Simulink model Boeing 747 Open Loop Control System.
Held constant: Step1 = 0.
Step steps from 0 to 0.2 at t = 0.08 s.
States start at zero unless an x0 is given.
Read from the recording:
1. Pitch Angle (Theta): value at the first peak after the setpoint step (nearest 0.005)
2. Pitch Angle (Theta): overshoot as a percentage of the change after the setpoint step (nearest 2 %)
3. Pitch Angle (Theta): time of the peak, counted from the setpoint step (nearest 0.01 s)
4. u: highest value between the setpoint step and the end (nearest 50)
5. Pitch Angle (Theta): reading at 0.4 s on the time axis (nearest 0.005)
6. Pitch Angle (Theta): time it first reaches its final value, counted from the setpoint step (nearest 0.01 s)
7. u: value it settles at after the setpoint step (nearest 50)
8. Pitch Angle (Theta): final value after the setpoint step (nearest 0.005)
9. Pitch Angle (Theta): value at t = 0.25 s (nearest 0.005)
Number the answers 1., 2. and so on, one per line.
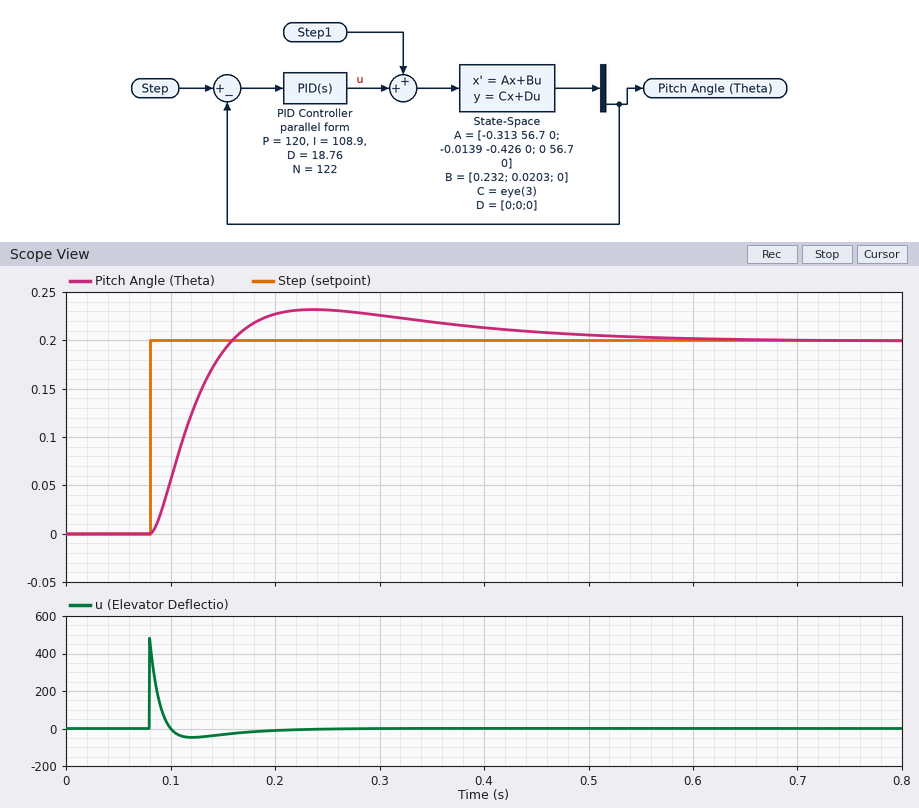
1. 0.230
2. 16 %
3. 0.16 s
4. 500
5. 0.215
6. 0.08 s
7. 0
8. 0.200
9. 0.230
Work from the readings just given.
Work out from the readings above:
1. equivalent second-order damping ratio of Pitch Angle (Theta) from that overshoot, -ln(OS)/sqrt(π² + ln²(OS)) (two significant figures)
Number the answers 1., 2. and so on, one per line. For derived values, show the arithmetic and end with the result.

1. ln(0.16) = -1.833; 1.833 / sqrt(9.870 + 3.358) = 0.50
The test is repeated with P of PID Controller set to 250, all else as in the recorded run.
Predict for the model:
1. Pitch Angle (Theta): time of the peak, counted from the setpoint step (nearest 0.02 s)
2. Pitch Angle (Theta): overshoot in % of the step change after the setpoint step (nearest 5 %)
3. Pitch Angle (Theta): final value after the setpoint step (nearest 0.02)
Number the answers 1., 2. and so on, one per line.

1. 0.12 s
2. 25 %
3. 0.20
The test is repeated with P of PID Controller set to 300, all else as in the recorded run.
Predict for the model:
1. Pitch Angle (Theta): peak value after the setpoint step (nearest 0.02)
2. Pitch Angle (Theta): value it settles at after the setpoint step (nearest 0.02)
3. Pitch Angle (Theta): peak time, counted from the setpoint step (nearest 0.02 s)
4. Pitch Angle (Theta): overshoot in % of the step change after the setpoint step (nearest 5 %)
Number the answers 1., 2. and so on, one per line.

1. 0.26
2. 0.20
3. 0.12 s
4. 30 %
